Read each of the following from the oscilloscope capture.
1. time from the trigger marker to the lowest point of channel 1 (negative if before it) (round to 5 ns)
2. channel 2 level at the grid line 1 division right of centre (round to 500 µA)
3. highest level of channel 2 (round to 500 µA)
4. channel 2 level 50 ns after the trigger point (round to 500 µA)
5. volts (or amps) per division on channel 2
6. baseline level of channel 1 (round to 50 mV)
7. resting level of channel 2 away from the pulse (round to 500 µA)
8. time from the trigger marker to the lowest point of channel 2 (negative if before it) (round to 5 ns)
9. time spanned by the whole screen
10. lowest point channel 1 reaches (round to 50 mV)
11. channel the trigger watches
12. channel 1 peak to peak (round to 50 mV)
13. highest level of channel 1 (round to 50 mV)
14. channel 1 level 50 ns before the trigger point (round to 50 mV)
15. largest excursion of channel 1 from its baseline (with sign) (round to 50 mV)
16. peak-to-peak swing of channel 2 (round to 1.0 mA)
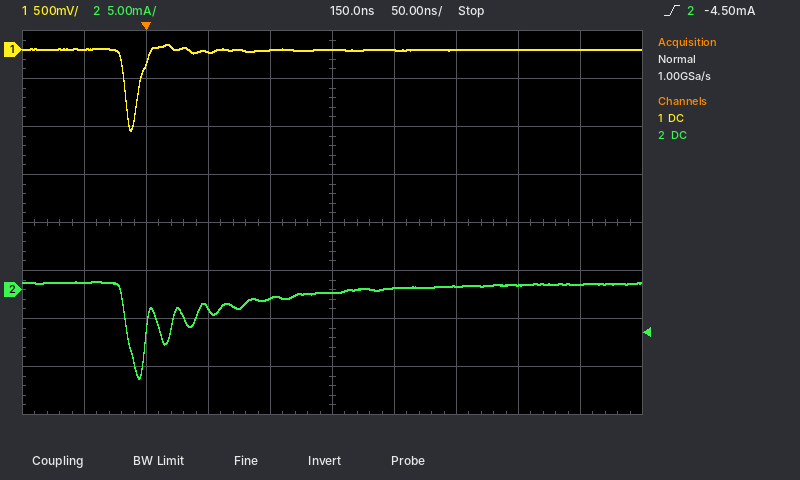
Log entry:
-10 ns
0.0 mA
1.0 mA
-2.0 mA
5 mA
0 mV
500 µA
-5 ns
500 ns
-850 mV
channel 2
900 mV
50 mV
0 mV
-850 mV
10.0 mA
